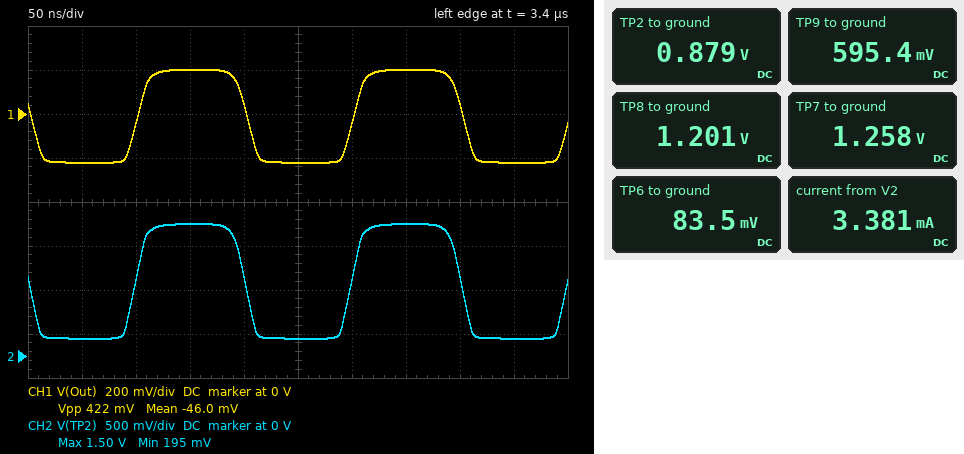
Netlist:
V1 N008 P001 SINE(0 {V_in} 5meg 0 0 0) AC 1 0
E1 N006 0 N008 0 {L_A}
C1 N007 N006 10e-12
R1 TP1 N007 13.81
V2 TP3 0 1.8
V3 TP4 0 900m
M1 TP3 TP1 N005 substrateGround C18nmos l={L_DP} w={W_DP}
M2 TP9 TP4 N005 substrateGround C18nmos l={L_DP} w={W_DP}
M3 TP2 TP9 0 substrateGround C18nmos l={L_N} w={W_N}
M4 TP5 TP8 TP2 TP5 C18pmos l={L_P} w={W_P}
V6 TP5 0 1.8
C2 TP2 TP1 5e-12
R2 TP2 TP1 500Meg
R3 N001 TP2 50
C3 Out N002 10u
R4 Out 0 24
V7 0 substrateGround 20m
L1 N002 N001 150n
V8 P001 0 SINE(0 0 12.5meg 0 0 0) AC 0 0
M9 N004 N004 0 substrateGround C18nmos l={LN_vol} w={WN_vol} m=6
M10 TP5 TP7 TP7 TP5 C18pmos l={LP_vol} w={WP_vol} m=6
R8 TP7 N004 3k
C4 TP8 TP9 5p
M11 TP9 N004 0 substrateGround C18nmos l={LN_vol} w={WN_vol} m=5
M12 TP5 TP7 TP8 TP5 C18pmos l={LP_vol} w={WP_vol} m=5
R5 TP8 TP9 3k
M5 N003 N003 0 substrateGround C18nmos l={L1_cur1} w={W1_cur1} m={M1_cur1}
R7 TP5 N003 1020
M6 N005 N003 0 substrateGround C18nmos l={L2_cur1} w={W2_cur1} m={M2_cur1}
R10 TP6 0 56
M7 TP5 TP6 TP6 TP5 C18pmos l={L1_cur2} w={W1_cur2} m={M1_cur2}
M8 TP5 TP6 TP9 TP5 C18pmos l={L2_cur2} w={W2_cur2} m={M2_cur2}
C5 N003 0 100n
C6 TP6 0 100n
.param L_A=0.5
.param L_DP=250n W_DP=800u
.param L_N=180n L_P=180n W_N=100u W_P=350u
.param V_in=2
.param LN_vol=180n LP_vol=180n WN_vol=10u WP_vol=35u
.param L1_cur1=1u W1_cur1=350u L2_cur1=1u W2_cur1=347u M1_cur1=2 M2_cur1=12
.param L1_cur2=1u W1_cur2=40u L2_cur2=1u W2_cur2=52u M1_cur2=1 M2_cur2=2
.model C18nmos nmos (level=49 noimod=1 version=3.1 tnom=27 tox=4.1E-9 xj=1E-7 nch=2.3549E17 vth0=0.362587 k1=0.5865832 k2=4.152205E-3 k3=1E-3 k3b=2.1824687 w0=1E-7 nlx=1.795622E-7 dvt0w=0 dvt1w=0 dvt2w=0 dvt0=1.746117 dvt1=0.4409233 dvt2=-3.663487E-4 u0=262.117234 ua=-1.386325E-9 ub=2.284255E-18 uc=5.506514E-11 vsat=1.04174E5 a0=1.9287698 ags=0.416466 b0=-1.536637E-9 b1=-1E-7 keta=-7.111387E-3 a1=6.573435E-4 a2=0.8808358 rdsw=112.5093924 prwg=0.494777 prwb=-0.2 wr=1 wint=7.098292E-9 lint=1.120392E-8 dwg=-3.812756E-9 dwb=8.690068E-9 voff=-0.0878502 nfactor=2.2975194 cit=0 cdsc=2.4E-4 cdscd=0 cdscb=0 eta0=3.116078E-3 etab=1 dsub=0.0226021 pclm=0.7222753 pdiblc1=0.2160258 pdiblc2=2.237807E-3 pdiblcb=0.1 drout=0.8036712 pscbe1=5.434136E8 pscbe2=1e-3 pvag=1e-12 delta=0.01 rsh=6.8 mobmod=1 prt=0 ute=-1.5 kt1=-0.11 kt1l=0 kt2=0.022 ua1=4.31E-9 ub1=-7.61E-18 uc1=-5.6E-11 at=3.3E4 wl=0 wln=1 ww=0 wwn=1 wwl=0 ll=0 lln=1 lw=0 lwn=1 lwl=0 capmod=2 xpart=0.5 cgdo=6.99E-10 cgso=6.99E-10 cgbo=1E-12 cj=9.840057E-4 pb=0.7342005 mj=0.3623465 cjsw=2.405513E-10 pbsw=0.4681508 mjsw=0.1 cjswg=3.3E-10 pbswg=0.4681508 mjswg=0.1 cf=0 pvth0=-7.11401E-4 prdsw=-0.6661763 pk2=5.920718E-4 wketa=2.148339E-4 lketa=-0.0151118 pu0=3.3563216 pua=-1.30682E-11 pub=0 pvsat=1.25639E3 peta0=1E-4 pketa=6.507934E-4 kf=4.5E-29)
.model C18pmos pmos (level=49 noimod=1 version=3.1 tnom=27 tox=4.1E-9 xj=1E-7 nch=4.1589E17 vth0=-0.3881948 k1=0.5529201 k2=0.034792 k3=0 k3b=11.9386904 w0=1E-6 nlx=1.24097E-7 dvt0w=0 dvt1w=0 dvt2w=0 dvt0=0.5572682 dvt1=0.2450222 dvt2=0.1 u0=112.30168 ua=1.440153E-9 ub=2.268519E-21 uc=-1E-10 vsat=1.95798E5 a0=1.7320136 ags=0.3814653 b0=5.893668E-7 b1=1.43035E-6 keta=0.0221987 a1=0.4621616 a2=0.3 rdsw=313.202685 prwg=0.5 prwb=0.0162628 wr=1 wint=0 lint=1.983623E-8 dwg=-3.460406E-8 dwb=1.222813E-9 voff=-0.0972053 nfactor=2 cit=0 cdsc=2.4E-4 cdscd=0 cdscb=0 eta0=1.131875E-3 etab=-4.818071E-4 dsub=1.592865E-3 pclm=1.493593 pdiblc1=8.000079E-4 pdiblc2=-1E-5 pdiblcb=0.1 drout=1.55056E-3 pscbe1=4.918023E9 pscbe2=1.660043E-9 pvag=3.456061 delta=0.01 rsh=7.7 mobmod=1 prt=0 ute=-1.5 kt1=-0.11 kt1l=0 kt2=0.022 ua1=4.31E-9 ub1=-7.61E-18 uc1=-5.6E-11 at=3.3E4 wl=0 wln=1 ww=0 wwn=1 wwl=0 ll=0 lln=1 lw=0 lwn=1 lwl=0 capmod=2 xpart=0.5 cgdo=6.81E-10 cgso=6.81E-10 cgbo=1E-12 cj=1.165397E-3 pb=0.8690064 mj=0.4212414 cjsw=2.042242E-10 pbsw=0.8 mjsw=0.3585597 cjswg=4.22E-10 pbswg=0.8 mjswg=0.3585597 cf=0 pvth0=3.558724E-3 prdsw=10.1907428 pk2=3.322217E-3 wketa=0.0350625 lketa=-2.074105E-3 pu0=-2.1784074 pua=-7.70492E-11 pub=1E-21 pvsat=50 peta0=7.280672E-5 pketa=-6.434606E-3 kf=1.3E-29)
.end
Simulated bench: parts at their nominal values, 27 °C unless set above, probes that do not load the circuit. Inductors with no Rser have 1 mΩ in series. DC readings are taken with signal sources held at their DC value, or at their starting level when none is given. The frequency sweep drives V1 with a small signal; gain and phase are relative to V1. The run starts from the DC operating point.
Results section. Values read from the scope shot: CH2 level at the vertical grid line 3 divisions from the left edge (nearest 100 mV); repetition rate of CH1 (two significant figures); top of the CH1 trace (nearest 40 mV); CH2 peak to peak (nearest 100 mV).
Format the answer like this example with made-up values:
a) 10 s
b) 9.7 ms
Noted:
a) 1.5 V
b) 5.0 MHz
c) 200 mV
d) 1.3 V
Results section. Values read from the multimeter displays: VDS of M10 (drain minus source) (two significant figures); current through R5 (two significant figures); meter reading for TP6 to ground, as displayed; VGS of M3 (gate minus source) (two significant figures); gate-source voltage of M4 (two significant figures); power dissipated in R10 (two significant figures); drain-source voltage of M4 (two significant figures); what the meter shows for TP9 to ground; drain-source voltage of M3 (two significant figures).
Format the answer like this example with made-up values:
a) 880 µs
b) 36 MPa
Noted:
a) 540 mV
b) 200 µA
c) 83.5 mV
d) 600 mV
e) 320 mV
f) 120 µW
g) 920 mV
h) 595.4 mV
i) 880 mV
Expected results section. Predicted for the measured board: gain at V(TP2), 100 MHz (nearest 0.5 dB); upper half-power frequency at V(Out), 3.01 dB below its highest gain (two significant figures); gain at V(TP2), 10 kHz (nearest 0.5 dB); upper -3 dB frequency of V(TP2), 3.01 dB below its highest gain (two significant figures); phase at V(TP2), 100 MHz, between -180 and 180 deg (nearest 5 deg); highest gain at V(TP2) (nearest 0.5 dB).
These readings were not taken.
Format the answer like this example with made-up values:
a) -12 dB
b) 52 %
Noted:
a) -0.5 dB
b) 77 MHz
c) -0.5 dB
d) 910 MHz
e) 170 deg
f) 9.0 dB
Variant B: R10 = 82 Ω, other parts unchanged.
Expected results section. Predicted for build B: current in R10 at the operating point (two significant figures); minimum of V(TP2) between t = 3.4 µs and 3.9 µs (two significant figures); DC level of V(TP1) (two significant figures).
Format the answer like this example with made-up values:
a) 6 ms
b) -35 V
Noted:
a) 1.4 mA
b) 200 mV
c) 890 mV
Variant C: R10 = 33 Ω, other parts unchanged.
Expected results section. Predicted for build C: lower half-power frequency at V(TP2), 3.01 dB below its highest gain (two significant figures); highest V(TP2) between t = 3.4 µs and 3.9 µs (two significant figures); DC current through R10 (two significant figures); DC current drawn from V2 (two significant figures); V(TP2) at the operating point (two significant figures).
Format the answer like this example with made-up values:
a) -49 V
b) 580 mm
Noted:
a) 540 MHz
b) 1.5 V
c) 1.6 mA
d) 3.2 mA
e) 870 mV
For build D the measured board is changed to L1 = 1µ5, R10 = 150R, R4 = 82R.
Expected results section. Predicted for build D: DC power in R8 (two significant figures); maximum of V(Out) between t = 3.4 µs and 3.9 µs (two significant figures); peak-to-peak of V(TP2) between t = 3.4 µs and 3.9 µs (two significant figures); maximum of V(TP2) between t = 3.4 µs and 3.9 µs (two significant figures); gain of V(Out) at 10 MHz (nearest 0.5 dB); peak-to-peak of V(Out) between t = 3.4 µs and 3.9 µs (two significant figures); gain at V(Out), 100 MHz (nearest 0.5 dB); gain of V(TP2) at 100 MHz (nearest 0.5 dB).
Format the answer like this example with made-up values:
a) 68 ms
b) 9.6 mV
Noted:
a) 170 µW
b) 450 mV
c) 1.6 V
d) 1.7 V
e) -6.0 dB
f) 930 mV
g) -21.0 dB
h) 0 dB
